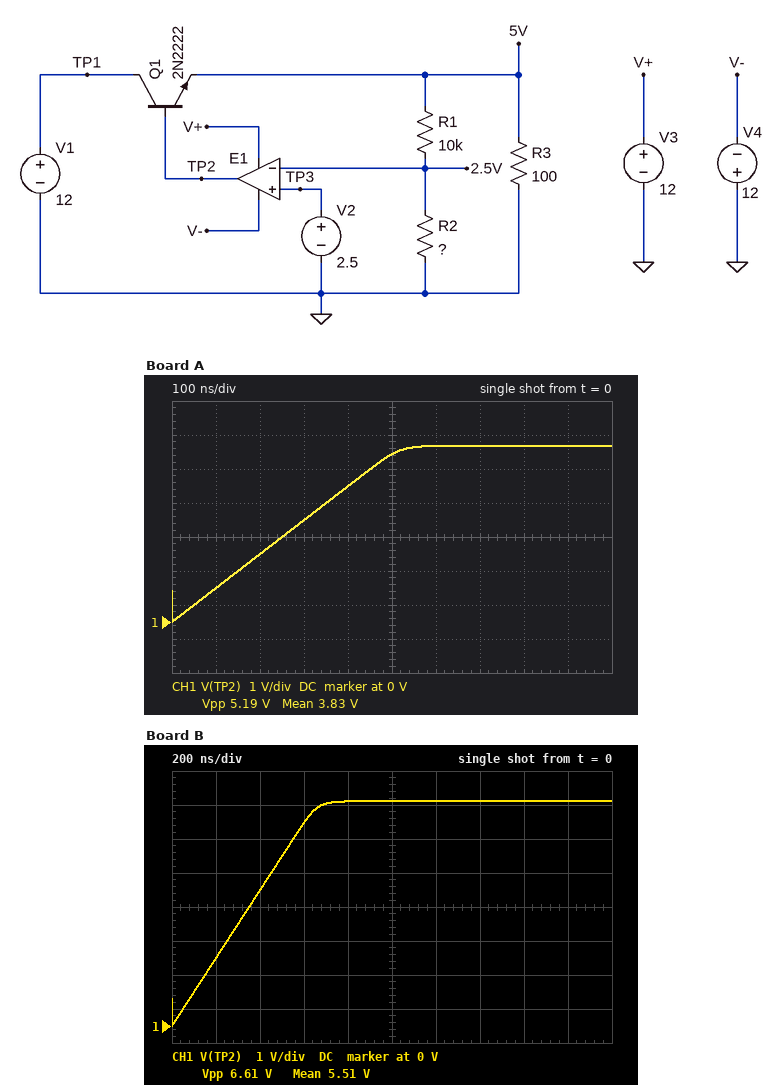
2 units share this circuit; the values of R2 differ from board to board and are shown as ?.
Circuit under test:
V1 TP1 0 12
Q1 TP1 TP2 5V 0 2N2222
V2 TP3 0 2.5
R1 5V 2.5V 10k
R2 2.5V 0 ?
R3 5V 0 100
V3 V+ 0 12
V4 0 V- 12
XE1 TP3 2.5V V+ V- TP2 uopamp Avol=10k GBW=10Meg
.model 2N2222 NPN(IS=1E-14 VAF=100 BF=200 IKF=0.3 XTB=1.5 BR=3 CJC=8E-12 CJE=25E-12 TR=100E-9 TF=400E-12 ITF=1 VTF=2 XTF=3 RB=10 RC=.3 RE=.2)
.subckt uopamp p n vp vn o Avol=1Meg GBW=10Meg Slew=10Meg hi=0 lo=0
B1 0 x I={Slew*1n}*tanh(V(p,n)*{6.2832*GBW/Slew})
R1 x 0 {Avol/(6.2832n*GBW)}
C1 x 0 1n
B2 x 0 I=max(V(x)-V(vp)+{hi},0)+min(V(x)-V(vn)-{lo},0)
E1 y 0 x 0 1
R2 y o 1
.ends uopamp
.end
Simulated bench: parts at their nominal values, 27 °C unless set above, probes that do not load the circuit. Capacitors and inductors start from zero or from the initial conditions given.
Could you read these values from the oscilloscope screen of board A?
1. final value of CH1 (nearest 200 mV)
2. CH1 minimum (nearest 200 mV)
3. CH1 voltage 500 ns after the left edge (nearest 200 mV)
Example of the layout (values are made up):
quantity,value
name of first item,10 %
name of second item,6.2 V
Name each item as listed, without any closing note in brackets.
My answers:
quantity,value
final value of CH1,5.2 V
CH1 minimum,0 V
CH1 voltage 500 ns after the left edge,5.0 V
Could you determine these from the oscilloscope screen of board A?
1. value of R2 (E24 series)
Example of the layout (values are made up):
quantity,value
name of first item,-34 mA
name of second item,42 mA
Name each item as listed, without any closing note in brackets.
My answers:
quantity,value
value of R2,13 kΩ
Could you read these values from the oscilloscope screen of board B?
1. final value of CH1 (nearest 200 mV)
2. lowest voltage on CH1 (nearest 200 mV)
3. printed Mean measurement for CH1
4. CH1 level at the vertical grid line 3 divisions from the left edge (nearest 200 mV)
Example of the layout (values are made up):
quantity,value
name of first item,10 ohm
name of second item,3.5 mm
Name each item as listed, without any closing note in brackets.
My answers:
quantity,value
final value of CH1,6.6 V
lowest voltage on CH1,0 V
printed Mean measurement for CH1,5.51 V
CH1 level at the vertical grid line 3 divisions from the left edge,6.0 V
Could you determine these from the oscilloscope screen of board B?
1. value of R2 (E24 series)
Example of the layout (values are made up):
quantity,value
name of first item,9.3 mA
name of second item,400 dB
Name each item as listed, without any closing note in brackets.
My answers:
quantity,value
value of R2,7.5 kΩ
